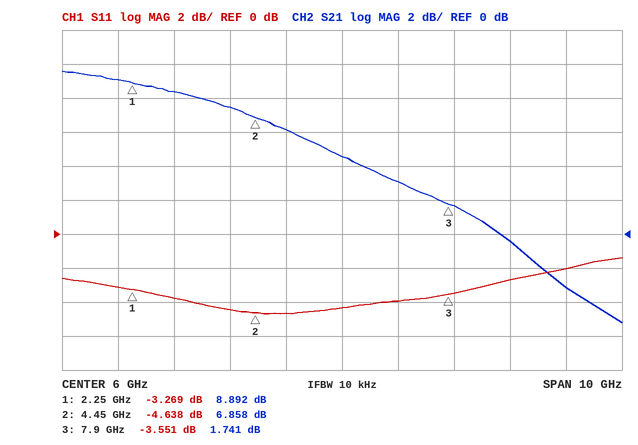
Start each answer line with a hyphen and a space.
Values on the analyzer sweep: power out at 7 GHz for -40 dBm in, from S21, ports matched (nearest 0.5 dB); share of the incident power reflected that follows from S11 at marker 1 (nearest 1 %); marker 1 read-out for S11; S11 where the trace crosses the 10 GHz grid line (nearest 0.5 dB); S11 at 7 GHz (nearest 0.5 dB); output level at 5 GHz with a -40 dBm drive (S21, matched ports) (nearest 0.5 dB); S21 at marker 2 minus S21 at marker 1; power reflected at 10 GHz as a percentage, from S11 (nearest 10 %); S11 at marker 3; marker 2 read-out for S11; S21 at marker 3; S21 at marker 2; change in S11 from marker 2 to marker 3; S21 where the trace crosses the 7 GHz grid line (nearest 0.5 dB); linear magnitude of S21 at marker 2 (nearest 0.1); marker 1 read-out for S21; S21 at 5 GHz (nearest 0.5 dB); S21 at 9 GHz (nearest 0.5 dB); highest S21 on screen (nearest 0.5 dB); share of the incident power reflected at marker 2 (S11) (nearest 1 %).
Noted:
- -37.0 dBm
- 47 %
- -3.269 dB
- -2.0 dB
- -4.0 dB
- -34.0 dBm
- -2.034 dB
- 60 %
- -3.551 dB
- -4.638 dB
- 1.741 dB
- 6.858 dB
- 1.087 dB
- 3.0 dB
- 2.2
- 8.892 dB
- 6.0 dB
- -0.5 dB
- 9.5 dB
- 34 %
